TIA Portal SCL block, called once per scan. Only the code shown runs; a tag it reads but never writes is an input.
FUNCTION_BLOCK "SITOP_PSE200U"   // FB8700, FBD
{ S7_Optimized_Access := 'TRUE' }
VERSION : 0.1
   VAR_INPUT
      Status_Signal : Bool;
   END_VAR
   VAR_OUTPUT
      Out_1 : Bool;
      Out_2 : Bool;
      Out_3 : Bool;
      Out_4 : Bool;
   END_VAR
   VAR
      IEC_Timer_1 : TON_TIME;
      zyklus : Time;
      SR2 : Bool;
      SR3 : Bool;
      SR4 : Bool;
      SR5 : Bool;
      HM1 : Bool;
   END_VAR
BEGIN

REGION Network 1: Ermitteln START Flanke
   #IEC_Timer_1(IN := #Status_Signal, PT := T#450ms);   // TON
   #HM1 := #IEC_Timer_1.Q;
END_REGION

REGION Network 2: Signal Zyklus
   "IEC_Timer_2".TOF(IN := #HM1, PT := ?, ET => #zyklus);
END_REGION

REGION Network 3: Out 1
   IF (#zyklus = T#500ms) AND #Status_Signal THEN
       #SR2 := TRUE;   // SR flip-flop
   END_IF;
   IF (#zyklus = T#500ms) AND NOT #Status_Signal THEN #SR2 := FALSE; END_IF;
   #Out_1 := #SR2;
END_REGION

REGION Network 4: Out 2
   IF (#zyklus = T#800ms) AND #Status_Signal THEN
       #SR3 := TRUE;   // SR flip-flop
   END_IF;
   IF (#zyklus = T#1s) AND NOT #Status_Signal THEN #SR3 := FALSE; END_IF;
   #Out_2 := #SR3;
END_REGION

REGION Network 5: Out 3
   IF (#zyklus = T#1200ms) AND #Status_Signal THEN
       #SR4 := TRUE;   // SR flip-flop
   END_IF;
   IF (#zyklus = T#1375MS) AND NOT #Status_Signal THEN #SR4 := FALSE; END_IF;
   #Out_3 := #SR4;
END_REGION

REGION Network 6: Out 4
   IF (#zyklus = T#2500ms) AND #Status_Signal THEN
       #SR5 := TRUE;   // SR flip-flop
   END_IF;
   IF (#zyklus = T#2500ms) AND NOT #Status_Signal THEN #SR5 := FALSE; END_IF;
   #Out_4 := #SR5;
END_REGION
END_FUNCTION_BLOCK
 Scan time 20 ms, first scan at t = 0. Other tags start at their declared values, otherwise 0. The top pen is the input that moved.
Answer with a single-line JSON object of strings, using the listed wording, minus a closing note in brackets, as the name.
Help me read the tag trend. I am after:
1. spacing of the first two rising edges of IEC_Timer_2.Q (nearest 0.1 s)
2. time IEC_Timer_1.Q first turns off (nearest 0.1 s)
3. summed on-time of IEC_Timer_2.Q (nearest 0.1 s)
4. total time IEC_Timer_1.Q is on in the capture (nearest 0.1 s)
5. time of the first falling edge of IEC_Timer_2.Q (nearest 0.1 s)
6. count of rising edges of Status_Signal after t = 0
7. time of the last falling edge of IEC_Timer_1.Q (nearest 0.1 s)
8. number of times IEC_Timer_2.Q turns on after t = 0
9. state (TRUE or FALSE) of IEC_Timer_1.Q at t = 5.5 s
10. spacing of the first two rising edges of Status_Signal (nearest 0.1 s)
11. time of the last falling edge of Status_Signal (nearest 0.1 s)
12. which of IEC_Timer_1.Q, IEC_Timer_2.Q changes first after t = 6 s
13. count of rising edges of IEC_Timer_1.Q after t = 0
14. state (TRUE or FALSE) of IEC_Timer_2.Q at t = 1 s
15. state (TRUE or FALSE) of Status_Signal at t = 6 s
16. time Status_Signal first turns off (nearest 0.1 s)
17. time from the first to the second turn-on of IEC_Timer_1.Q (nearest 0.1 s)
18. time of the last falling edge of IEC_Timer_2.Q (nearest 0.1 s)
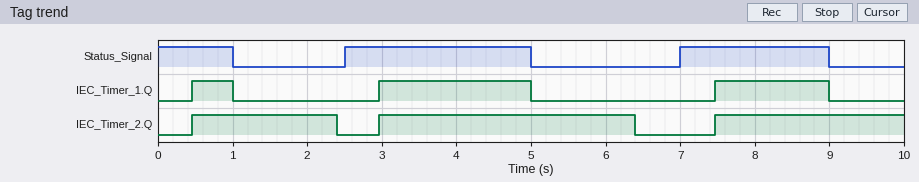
{"spacing of the first two rising edges of IEC_Timer_2.Q": "2.5 s", "time IEC_Timer_1.Q first turns off": "1.0 s", "summed on-time of IEC_Timer_2.Q": "7.9 s", "total time IEC_Timer_1.Q is on in the capture": "4.1 s", "time of the first falling edge of IEC_Timer_2.Q": "2.4 s", "count of rising edges of Status_Signal after t = 0": "2", "time of the last falling edge of IEC_Timer_1.Q": "9.0 s", "number of times IEC_Timer_2.Q turns on after t = 0": "3", "state (TRUE or FALSE) of IEC_Timer_1.Q at t = 5.5 s": "FALSE", "spacing of the first two rising edges of Status_Signal": "4.5 s", "time of the last falling edge of Status_Signal": "9.0 s", "which of IEC_Timer_1.Q, IEC_Timer_2.Q changes first after t = 6 s": "IEC_Timer_2.Q", "count of rising edges of IEC_Timer_1.Q after t = 0": "3", "state (TRUE or FALSE) of IEC_Timer_2.Q at t = 1 s": "TRUE", "state (TRUE or FALSE) of Status_Signal at t = 6 s": "FALSE", "time Status_Signal first turns off": "1.0 s", "time from the first to the second turn-on of IEC_Timer_1.Q": "2.5 s", "time of the last falling edge of IEC_Timer_2.Q": "6.4 s"}
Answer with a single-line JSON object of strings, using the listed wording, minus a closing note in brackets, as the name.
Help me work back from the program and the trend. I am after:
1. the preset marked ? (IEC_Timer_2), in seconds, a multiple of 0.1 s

{"the preset marked ? (IEC_Timer_2), in seconds, a multiple of 0.1 s": "1.4 s"}
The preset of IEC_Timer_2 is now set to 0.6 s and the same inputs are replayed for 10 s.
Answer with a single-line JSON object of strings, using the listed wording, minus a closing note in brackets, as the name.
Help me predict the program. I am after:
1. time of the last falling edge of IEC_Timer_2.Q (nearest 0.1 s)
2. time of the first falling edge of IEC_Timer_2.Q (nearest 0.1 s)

{"time of the last falling edge of IEC_Timer_2.Q": "9.6 s", "time of the first falling edge of IEC_Timer_2.Q": "1.6 s"}
